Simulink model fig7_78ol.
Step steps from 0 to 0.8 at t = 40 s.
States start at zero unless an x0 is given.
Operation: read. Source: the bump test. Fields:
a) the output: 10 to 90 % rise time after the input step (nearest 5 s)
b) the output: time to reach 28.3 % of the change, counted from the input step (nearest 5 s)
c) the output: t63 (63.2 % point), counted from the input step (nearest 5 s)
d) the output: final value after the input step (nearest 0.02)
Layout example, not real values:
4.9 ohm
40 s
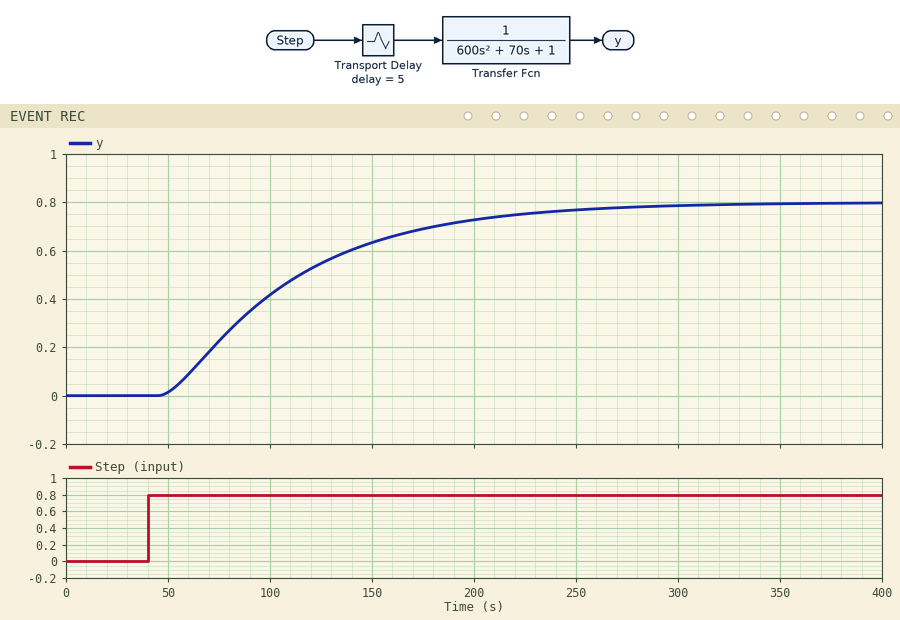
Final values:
135 s
35 s
75 s
0.80
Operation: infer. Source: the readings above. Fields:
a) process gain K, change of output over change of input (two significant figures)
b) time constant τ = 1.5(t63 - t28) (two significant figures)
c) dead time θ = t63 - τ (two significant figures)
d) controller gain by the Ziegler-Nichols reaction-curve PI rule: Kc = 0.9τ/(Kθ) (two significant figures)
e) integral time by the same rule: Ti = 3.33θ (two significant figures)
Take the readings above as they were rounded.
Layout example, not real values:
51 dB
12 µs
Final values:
1.0
60 s
15 s
3.6
50 s
